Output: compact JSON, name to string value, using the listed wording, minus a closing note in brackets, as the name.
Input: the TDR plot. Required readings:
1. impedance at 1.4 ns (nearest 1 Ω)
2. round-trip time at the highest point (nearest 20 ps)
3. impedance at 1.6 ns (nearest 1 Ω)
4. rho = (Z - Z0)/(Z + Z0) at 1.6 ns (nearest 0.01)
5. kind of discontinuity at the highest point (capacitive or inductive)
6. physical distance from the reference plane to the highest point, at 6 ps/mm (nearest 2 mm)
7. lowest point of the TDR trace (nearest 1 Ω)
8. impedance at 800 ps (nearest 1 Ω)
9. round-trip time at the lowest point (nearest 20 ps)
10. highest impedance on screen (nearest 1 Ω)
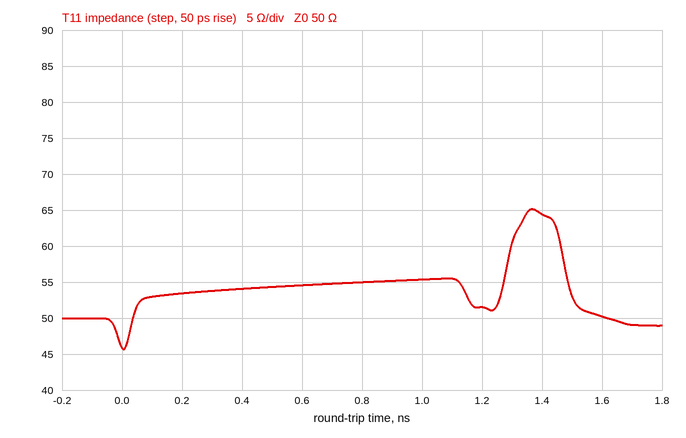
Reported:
{"impedance at 1.4 ns": "64 Ω", "round-trip time at the highest point": "1.36 ns", "impedance at 1.6 ns": "50 Ω", "rho = (Z - Z0)/(Z + Z0) at 1.6 ns": "0.00", "kind of discontinuity at the highest point": "inductive", "physical distance from the reference plane to the highest point, at 6 ps/mm": "114 mm", "lowest point of the TDR trace": "46 Ω", "impedance at 800 ps": "55 Ω", "round-trip time at the lowest point": "0 ps", "highest impedance on screen": "65 Ω"}
